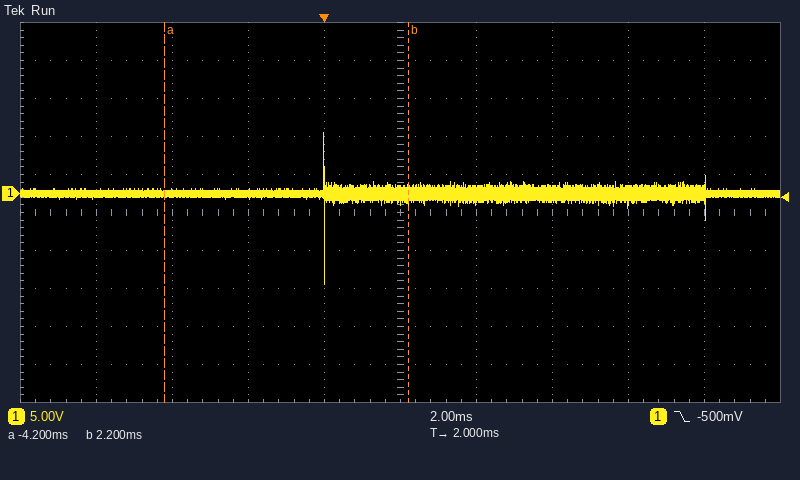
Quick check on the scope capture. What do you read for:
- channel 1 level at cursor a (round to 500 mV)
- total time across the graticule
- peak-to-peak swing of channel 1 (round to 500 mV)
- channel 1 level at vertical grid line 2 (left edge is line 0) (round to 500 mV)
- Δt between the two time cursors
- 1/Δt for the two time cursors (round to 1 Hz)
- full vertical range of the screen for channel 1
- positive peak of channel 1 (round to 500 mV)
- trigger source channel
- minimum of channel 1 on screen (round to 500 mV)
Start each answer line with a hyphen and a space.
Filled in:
- 0.0 V
- 20 ms
- 20.0 V
- 0.0 V
- 6.4 ms
- 156 Hz
- 50 V
- 8.0 V
- channel 1
- -12.0 V
